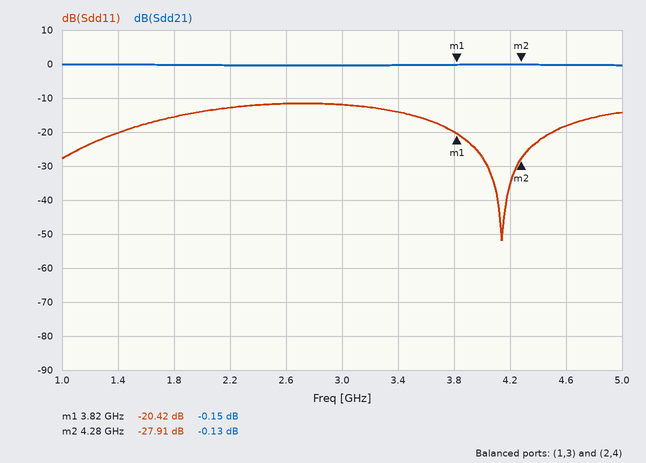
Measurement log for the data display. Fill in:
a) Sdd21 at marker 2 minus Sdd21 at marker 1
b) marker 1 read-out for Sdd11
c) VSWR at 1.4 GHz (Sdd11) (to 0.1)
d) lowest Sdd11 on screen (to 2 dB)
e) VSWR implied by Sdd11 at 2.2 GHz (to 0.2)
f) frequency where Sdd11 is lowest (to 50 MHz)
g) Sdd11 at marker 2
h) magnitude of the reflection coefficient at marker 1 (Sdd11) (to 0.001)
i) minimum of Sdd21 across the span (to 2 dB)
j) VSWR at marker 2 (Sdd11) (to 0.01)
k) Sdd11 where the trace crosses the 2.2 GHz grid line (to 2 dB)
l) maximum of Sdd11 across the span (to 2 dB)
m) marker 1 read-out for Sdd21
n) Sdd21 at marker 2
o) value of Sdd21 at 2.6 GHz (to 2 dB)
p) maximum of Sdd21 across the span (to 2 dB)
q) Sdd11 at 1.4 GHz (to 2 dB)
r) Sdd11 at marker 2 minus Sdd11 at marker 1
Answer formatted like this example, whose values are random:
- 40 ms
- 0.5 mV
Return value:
- 0.02 dB
- -20.42 dB
- 1.2
- -52 dB
- 1.6
- 4.15 GHz
- -27.91 dB
- 0.095
- 0 dB
- 1.08
- -12 dB
- -12 dB
- -0.15 dB
- -0.13 dB
- 0 dB
- 0 dB
- -20 dB
- -7.49 dB
